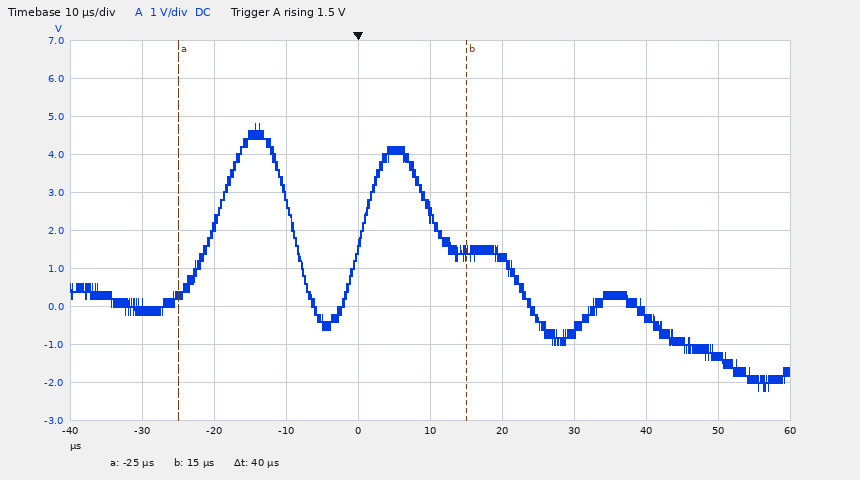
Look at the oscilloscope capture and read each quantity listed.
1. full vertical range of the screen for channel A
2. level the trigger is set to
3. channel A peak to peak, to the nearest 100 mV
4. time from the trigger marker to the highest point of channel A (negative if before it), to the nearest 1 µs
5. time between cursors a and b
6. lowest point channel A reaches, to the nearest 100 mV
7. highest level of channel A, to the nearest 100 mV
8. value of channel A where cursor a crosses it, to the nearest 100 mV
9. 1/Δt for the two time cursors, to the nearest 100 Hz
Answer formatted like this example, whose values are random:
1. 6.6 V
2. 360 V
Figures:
1. 10 V
2. 1.5 V
3. 7.0 V
4. -14 µs
5. 40 µs
6. -2.2 V
7. 4.8 V
8. 300 mV
9. 25.0 kHz
